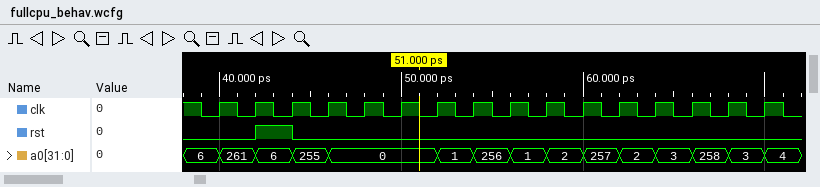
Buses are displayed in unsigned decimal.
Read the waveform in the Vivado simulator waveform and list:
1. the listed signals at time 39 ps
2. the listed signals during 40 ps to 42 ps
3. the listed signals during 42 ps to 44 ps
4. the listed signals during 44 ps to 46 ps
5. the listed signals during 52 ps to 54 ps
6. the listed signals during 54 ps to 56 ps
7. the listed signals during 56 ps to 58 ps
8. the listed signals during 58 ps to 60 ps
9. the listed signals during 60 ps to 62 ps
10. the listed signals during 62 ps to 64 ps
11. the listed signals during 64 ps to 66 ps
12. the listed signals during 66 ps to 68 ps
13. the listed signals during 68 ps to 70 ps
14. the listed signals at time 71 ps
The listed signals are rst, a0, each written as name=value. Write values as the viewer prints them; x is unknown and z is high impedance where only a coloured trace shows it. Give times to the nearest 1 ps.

rst=0, a0=6
rst=0, a0=261
rst=1, a0=6
rst=0, a0=255
rst=0, a0=1
rst=0, a0=256
rst=0, a0=1
rst=0, a0=2
rst=0, a0=257
rst=0, a0=2
rst=0, a0=3
rst=0, a0=258
rst=0, a0=3
rst=0, a0=4
